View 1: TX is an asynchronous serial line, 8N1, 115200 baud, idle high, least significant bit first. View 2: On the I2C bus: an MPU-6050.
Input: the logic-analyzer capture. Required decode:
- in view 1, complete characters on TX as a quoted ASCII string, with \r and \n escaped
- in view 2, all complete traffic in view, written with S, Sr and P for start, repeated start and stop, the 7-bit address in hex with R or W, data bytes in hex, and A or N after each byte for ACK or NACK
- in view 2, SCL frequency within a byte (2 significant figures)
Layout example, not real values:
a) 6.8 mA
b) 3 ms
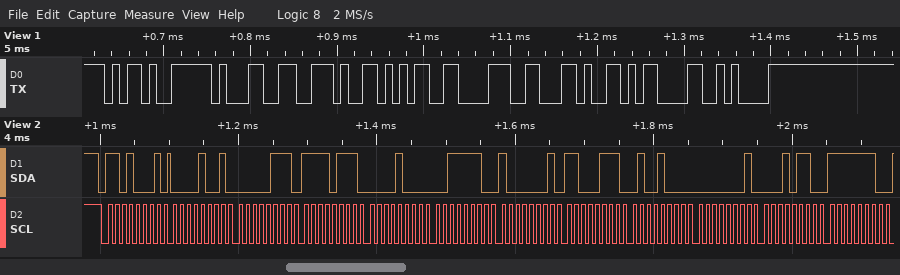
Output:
a) "-1.58,\r\n"
b) S 68R A 09 A 07 A F7 A 08 A 3E A 81 A C7 A 48 A 01 A 16 A FE A
c) 100 kHz
